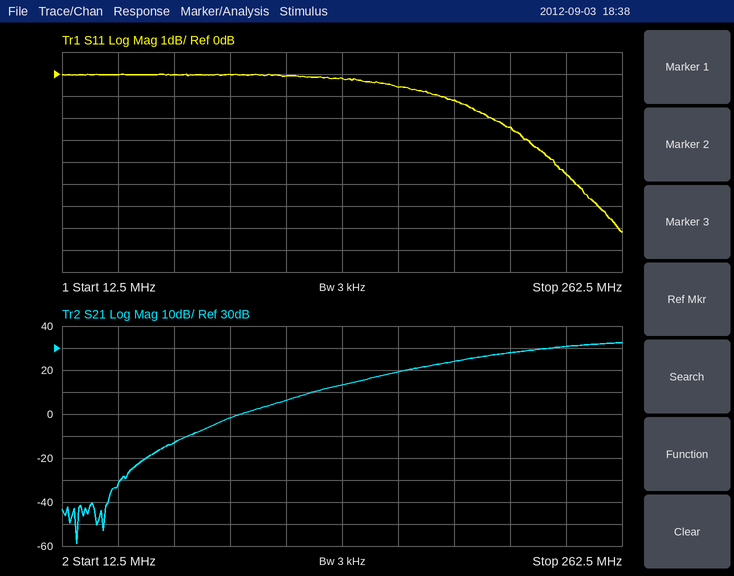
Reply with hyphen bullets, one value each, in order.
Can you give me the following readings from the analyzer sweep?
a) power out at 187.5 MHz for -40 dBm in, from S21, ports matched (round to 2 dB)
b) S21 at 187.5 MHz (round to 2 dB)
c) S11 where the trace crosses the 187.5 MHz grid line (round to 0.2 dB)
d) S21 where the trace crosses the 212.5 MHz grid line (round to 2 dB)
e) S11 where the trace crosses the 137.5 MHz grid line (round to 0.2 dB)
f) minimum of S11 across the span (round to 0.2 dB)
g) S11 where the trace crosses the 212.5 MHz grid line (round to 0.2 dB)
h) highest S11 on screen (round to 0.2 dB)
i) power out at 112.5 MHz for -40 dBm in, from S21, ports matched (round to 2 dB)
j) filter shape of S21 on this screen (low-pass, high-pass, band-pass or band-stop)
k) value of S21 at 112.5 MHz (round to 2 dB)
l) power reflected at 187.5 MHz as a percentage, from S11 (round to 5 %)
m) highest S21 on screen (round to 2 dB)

- -16 dBm
- 24 dB
- -1.2 dB
- 28 dB
- -0.2 dB
- -7.2 dB
- -2.4 dB
- 0.0 dB
- -34 dBm
- high-pass
- 6 dB
- 75 %
- 32 dB
